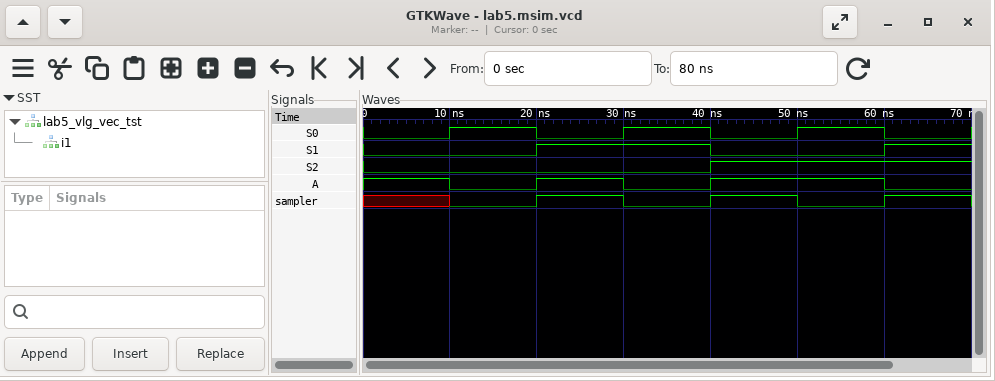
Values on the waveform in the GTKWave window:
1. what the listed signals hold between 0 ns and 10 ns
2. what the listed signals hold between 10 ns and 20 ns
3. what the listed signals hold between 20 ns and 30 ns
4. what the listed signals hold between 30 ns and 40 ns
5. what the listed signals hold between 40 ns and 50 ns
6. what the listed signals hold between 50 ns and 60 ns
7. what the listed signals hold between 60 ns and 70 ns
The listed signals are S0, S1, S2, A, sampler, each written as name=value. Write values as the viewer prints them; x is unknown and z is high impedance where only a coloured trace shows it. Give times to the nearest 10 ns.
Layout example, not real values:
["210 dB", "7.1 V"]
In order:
["S0=0, S1=0, S2=0, A=1, sampler=x", "S0=1, S1=0, S2=0, A=0, sampler=0", "S0=0, S1=1, S2=0, A=1, sampler=1", "S0=1, S1=1, S2=0, A=0, sampler=0", "S0=0, S1=0, S2=1, A=1, sampler=1", "S0=1, S1=0, S2=1, A=1, sampler=0", "S0=0, S1=1, S2=1, A=0, sampler=1"]
